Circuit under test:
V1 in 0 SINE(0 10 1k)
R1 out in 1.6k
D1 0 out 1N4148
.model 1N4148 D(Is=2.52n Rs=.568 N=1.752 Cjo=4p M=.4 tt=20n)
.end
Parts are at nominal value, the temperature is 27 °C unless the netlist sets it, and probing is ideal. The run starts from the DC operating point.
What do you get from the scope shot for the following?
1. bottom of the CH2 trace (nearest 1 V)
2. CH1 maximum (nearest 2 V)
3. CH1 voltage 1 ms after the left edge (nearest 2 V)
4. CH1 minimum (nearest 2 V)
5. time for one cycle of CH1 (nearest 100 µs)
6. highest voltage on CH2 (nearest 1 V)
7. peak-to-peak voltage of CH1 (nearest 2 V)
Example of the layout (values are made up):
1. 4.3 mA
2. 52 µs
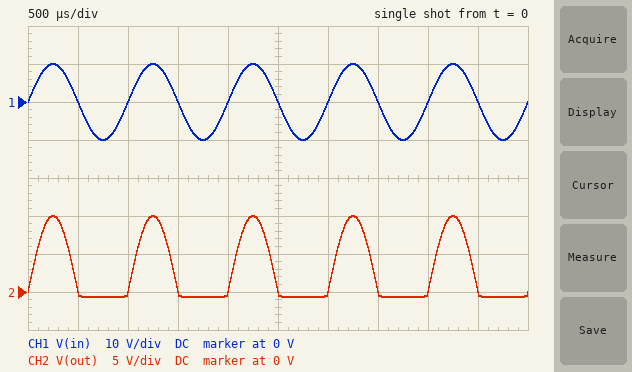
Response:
1. -1 V
2. 10 V
3. 0 V
4. -10 V
5. 1.0 ms
6. 10 V
7. 20 V
